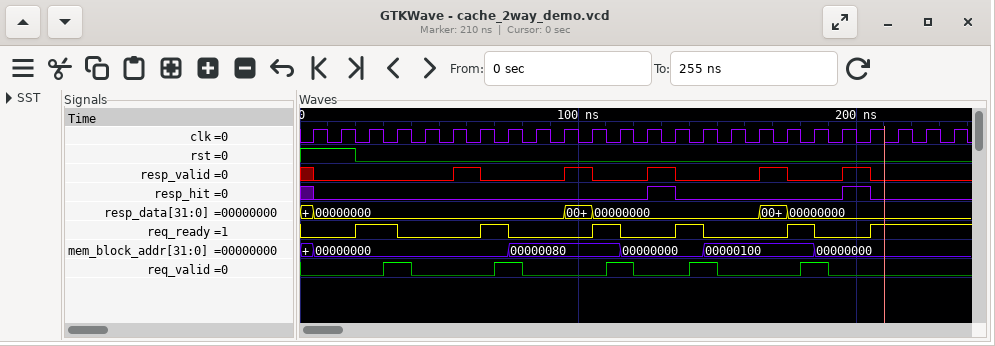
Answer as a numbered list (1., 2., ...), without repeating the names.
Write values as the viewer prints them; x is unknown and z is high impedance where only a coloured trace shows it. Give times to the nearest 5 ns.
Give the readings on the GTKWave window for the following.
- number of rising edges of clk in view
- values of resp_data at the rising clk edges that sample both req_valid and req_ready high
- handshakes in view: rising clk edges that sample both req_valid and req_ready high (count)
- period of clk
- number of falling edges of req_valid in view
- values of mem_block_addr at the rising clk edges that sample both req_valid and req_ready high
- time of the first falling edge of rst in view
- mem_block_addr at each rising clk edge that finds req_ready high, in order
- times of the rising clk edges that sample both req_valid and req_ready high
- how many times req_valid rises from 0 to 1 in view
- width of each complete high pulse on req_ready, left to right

1. 24
2. 00000000, 00000000, 00000000, 00000000, 00000000
3. 5
4. 10 ns
5. 5
6. 00000000, 00000000, 00000080, 00000000, 00000100
7. 20 ns
8. 00000000, 00000000, 00000000, 00000080, 00000000, 00000100, 00000000, 00000000, 00000000
9. 35 ns, 75 ns, 115 ns, 145 ns, 185 ns
10. 5
11. 15 ns, 10 ns, 10 ns, 10 ns, 10 ns
